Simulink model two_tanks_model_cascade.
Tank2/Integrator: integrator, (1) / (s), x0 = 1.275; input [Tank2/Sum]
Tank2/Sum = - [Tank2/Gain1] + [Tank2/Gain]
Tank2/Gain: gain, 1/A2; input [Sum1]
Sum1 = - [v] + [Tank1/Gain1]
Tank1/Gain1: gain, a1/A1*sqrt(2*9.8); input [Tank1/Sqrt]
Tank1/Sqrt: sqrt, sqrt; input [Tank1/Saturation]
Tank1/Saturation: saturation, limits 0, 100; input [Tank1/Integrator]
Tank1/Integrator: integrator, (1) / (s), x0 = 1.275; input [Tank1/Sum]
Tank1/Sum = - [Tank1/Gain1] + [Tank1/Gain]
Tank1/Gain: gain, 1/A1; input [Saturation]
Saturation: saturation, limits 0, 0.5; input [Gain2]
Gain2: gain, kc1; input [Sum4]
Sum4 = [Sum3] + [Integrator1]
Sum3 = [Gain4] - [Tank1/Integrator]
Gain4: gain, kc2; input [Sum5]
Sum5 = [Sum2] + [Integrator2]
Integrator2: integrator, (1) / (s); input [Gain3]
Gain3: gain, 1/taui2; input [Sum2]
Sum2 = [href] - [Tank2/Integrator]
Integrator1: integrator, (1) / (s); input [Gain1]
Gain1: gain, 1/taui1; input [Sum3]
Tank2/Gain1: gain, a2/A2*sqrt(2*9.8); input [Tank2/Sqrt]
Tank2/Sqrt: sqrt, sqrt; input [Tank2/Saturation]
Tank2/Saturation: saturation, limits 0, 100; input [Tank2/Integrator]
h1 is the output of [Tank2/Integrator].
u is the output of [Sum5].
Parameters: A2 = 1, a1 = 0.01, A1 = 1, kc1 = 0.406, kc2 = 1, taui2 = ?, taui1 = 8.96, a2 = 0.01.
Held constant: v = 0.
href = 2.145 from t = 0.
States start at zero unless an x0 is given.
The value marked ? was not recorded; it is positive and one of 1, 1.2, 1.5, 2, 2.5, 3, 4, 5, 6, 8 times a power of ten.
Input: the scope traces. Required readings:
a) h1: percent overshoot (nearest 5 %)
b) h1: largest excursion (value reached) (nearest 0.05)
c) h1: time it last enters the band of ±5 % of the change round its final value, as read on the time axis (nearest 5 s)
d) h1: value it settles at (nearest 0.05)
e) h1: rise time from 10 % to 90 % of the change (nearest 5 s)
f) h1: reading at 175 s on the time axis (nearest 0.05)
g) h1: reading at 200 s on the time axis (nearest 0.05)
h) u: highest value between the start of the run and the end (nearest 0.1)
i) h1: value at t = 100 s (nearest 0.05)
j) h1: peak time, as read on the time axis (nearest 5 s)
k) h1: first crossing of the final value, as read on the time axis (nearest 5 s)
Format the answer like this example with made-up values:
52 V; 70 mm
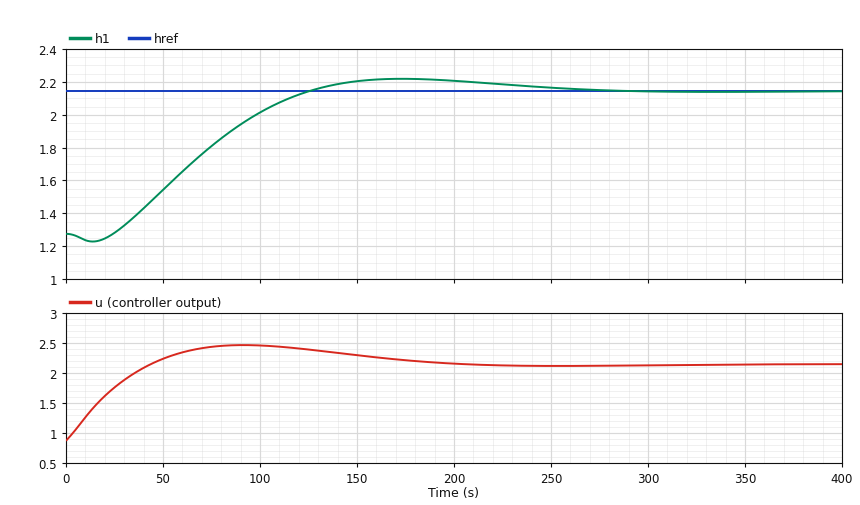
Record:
10 %; 2.20; 220 s; 2.15; 75 s; 2.20; 2.20; 2.5; 2.00; 175 s; 125 s
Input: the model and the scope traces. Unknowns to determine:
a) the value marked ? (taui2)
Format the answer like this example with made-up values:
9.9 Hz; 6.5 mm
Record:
25
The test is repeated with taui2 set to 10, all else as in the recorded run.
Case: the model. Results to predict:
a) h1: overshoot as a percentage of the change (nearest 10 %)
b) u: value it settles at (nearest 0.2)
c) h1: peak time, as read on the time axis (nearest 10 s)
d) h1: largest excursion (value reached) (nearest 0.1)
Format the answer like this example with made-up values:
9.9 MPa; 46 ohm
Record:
30 %; 2.2; 90 s; 2.4
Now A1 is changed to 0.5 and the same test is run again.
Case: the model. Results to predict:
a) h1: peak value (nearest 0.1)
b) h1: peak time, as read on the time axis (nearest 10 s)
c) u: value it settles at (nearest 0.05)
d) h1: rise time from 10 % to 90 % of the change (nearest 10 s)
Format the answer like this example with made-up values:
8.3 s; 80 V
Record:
2.2; 70 s; 0.55; 40 s
